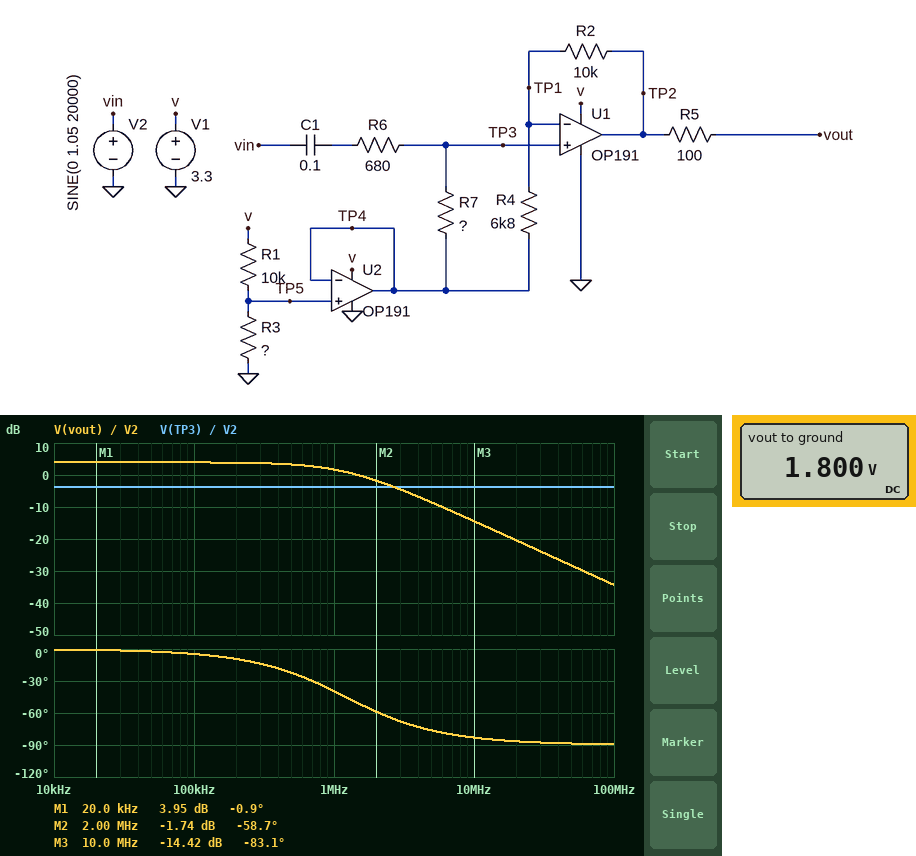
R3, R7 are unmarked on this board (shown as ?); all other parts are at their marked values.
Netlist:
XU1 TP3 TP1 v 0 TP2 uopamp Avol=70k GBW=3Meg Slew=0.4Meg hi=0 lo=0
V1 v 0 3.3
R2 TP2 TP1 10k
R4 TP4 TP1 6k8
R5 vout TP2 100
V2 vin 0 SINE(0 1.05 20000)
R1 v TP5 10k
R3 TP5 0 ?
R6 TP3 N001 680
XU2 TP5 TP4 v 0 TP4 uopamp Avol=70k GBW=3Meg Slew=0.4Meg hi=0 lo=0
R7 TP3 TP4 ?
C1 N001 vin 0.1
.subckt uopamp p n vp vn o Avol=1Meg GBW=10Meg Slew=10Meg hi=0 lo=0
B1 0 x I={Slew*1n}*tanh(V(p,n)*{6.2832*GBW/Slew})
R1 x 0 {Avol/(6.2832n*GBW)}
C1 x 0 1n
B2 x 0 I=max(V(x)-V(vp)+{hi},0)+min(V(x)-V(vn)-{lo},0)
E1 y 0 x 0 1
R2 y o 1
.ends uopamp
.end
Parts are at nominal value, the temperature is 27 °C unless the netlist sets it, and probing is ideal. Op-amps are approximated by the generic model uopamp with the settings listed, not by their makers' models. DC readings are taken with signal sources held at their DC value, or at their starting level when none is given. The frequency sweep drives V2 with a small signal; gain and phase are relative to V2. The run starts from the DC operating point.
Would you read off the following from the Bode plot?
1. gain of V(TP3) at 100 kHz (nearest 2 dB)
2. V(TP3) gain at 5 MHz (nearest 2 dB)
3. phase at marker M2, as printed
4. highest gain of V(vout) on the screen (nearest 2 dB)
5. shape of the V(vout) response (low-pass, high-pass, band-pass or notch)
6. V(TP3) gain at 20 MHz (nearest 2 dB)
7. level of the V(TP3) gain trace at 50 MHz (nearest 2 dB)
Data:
-4 dB
-4 dB
-58.7 deg
4 dB
low-pass
-4 dB
-4 dB
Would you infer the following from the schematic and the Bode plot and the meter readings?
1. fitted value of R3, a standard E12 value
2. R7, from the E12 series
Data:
12 kΩ
1.2 kΩ
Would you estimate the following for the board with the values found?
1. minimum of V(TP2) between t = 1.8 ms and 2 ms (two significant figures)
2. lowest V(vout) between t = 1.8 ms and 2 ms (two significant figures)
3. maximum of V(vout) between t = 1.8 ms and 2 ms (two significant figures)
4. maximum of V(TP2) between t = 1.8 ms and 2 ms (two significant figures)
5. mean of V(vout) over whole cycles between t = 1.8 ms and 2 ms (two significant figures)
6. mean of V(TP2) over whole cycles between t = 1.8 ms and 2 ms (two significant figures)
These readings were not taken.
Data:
140 mV
140 mV
3.3 V
3.3 V
1.8 V
1.8 V
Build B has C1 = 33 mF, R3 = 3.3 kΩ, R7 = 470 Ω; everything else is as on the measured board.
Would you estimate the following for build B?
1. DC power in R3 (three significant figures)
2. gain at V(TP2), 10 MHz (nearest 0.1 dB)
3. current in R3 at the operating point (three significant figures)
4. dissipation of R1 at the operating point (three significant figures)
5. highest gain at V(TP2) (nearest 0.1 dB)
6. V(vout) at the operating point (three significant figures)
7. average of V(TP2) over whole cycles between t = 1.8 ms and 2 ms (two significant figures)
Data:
203 µW
-18.3 dB
248 µA
616 µW
0.1 dB
819 mV
850 mV
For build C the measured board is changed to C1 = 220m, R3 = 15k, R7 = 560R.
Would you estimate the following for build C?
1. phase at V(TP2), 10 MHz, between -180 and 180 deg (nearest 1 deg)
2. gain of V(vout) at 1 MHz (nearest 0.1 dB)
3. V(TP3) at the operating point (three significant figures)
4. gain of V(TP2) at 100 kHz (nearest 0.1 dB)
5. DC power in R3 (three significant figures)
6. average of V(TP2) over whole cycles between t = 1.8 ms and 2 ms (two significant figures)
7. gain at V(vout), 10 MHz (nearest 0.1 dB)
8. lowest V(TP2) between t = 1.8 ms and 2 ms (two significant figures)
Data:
-83 deg
-1.3 dB
1.98 V
0.9 dB
261 µW
2.0 V
-17.4 dB
810 mV
